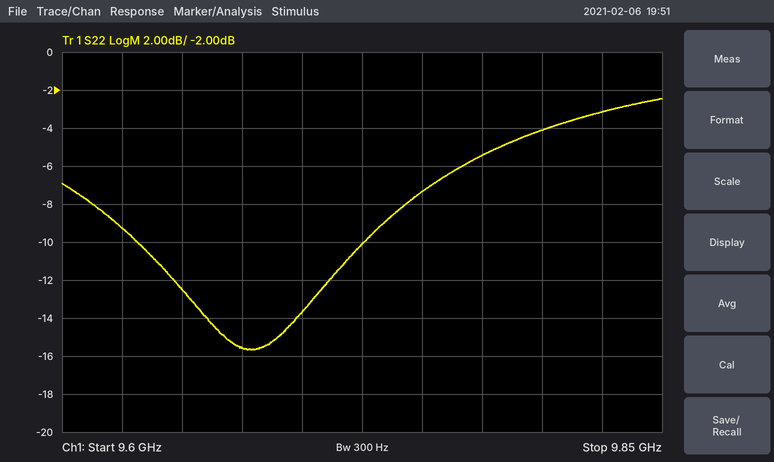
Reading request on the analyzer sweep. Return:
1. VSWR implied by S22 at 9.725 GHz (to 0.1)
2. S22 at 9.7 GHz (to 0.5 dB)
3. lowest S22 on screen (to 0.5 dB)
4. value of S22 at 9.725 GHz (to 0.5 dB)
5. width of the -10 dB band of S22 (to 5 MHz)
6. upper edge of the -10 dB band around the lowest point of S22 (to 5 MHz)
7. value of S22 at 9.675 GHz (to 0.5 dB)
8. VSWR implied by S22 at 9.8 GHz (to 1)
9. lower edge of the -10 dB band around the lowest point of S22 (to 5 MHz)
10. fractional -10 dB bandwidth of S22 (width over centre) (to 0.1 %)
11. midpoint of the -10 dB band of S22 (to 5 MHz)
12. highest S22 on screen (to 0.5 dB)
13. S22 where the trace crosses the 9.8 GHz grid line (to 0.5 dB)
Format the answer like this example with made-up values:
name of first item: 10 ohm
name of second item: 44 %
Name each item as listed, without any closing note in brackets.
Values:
VSWR implied by S22 at 9.725 GHz: 1.9
S22 at 9.7 GHz: -13.5 dB
lowest S22 on screen: -15.5 dB
value of S22 at 9.725 GHz: -10.0 dB
width of the -10 dB band of S22: 95 MHz
upper edge of the -10 dB band around the lowest point of S22: 9.725 GHz
value of S22 at 9.675 GHz: -15.5 dB
VSWR implied by S22 at 9.8 GHz: 4
lower edge of the -10 dB band around the lowest point of S22: 9.630 GHz
fractional -10 dB bandwidth of S22 (width over centre): 1.0 %
midpoint of the -10 dB band of S22: 9.680 GHz
highest S22 on screen: -2.5 dB
S22 where the trace crosses the 9.8 GHz grid line: -4.0 dB
